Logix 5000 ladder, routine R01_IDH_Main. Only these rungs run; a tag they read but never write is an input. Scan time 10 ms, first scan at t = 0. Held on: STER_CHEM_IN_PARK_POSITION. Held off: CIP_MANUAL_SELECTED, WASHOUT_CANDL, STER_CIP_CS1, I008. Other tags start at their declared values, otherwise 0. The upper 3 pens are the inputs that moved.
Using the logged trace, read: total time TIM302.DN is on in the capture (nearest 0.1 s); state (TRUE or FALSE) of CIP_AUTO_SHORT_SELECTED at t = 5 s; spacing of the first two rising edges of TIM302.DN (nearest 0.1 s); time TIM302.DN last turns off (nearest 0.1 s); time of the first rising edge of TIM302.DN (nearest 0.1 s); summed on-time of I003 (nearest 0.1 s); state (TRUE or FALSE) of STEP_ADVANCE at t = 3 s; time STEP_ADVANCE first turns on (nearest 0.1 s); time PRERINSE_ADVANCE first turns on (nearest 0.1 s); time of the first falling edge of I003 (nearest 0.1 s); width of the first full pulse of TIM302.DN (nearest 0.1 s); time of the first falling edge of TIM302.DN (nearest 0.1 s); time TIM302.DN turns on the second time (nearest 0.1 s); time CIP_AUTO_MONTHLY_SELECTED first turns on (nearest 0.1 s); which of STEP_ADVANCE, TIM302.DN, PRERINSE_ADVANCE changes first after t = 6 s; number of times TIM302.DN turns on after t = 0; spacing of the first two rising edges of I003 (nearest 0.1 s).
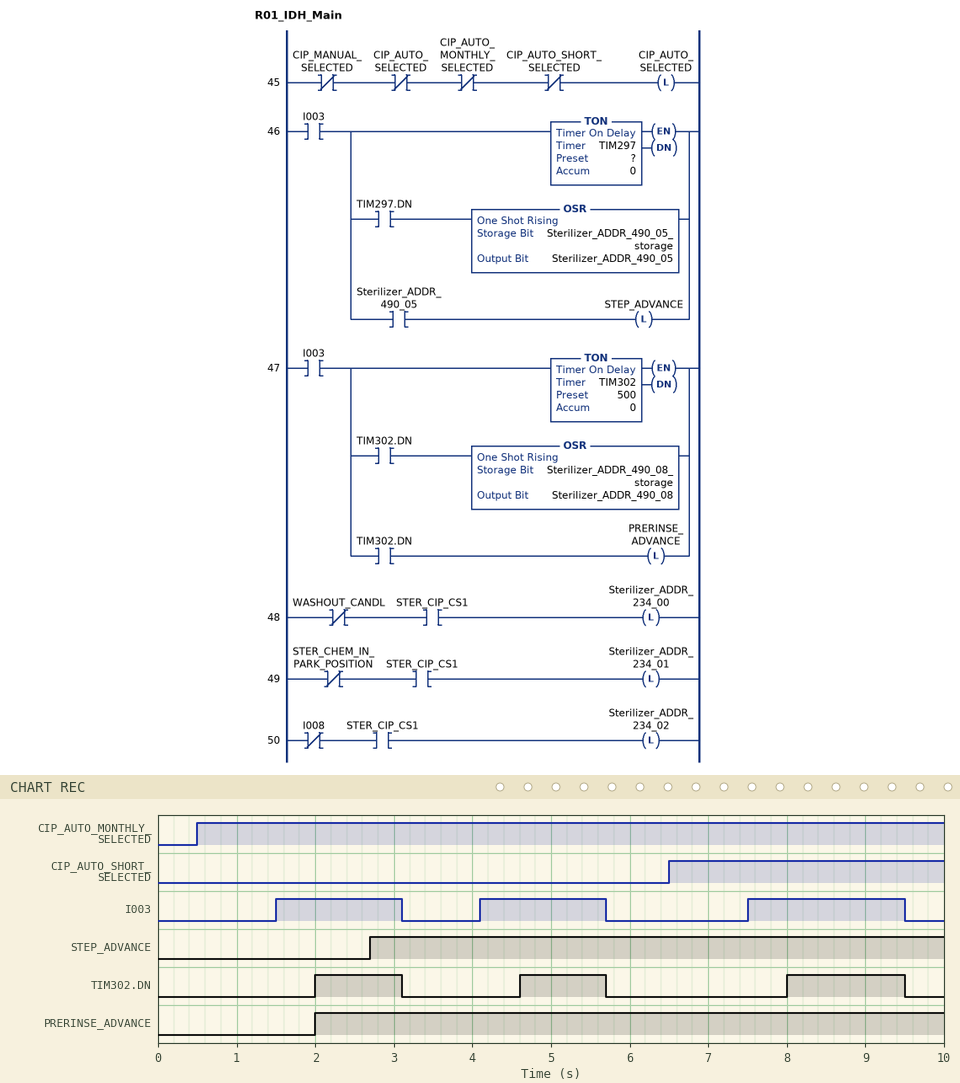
3.7 s
FALSE
2.6 s
9.5 s
2.0 s
5.2 s
TRUE
2.7 s
2.0 s
3.1 s
1.1 s
3.1 s
4.6 s
0.5 s
TIM302.DN
3
2.6 s
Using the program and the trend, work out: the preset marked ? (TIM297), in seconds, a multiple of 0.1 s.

1.2 s
